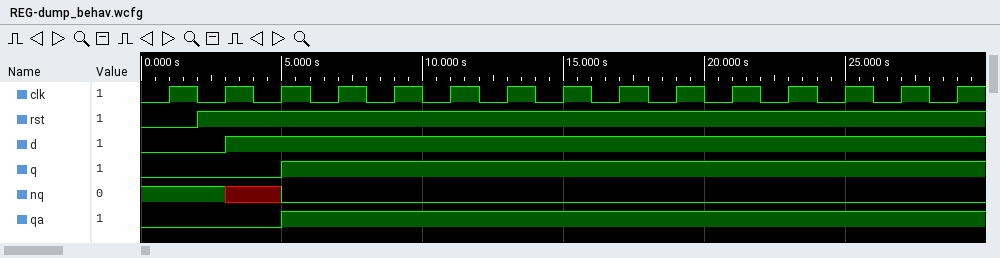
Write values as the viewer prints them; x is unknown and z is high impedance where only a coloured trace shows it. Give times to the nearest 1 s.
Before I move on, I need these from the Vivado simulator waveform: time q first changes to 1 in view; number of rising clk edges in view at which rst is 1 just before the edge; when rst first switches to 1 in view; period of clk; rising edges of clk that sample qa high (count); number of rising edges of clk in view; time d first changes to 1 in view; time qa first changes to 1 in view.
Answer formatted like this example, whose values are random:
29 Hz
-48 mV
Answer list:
5 s
14
2 s
2 s
12
15
3 s
5 s
